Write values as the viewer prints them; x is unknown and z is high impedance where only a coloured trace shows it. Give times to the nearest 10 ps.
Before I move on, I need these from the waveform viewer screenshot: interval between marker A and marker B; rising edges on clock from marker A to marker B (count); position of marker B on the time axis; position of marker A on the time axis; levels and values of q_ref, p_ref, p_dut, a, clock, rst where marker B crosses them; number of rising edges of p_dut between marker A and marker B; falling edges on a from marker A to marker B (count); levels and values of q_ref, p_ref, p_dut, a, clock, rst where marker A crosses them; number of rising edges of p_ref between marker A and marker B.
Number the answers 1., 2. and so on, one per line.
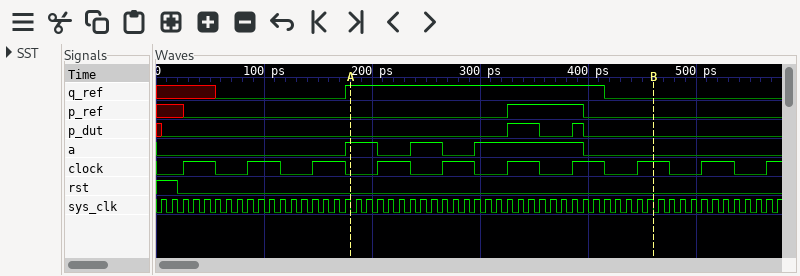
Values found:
1. 280 ps
2. 5
3. 460 ps
4. 180 ps
5. q_ref=0, p_ref=0, p_dut=0, a=0, clock=1, rst=0
6. 2
7. 3
8. q_ref=1, p_ref=0, p_dut=0, a=1, clock=0, rst=0
9. 1
